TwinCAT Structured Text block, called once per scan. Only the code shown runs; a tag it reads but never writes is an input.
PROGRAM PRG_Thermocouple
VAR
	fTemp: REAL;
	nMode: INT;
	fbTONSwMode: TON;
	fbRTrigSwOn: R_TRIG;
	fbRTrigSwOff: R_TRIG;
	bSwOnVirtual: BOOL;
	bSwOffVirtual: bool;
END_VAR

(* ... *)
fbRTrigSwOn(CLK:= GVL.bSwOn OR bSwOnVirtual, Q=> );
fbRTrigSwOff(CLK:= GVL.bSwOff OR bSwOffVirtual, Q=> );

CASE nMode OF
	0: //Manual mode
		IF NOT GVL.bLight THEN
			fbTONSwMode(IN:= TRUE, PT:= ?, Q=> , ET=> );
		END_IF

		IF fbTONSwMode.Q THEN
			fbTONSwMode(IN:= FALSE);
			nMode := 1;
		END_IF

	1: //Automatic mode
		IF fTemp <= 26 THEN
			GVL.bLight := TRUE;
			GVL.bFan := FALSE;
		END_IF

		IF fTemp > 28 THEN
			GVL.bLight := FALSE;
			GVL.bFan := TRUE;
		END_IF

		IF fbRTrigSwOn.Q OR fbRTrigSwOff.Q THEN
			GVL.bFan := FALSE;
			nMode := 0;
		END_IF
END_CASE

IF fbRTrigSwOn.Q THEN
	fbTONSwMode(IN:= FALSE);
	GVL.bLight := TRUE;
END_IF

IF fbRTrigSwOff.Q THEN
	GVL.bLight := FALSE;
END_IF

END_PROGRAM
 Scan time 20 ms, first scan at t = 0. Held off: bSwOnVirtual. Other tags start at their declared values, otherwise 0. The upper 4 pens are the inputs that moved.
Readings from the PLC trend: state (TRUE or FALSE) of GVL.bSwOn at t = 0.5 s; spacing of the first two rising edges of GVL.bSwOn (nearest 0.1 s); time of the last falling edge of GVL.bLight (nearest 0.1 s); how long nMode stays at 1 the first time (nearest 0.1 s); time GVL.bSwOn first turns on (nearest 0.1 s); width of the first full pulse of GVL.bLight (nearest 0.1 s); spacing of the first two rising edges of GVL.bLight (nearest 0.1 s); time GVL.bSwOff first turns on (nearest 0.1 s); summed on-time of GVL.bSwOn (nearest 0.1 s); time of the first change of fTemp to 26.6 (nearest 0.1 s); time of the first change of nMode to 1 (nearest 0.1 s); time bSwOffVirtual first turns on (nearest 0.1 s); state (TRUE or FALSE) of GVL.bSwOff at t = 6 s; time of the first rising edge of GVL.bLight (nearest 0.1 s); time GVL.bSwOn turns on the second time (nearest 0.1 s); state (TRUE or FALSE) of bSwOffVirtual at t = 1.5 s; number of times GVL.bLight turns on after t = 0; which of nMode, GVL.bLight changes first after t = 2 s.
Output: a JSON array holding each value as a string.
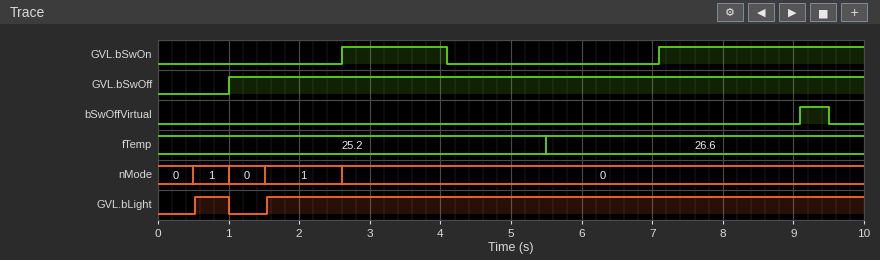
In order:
["FALSE", "4.5 s", "1.0 s", "0.5 s", "2.6 s", "0.5 s", "1.0 s", "1.0 s", "4.4 s", "5.5 s", "0.5 s", "9.1 s", "TRUE", "0.5 s", "7.1 s", "FALSE", "2", "nMode"]
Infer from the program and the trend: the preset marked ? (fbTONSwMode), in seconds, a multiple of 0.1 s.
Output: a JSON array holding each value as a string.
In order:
["0.5 s"]
